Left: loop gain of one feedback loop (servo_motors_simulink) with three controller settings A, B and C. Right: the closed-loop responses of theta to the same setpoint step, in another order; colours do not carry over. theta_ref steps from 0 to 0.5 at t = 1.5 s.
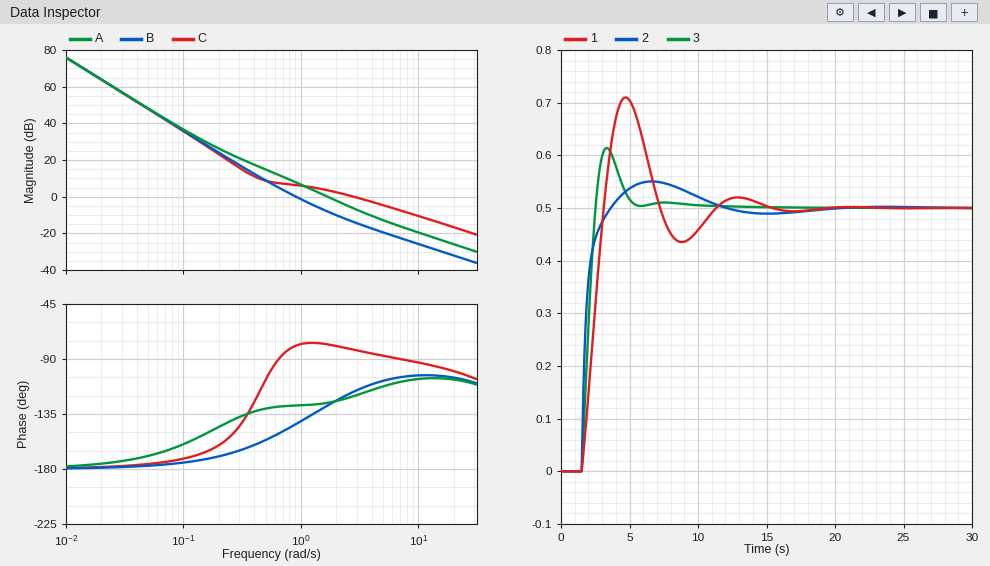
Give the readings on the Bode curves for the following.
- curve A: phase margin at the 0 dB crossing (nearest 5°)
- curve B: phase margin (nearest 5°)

55°
35°
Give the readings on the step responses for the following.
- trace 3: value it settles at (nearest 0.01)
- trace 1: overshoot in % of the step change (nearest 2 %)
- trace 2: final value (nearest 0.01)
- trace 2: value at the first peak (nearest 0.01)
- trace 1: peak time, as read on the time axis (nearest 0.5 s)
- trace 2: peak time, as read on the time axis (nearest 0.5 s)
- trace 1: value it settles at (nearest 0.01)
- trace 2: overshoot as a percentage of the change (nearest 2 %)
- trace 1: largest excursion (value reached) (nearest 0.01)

0.50
42 %
0.50
0.55
4.5 s
6.5 s
0.50
10 %
0.71
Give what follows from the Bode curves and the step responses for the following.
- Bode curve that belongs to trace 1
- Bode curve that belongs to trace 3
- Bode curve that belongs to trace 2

B
A
C
